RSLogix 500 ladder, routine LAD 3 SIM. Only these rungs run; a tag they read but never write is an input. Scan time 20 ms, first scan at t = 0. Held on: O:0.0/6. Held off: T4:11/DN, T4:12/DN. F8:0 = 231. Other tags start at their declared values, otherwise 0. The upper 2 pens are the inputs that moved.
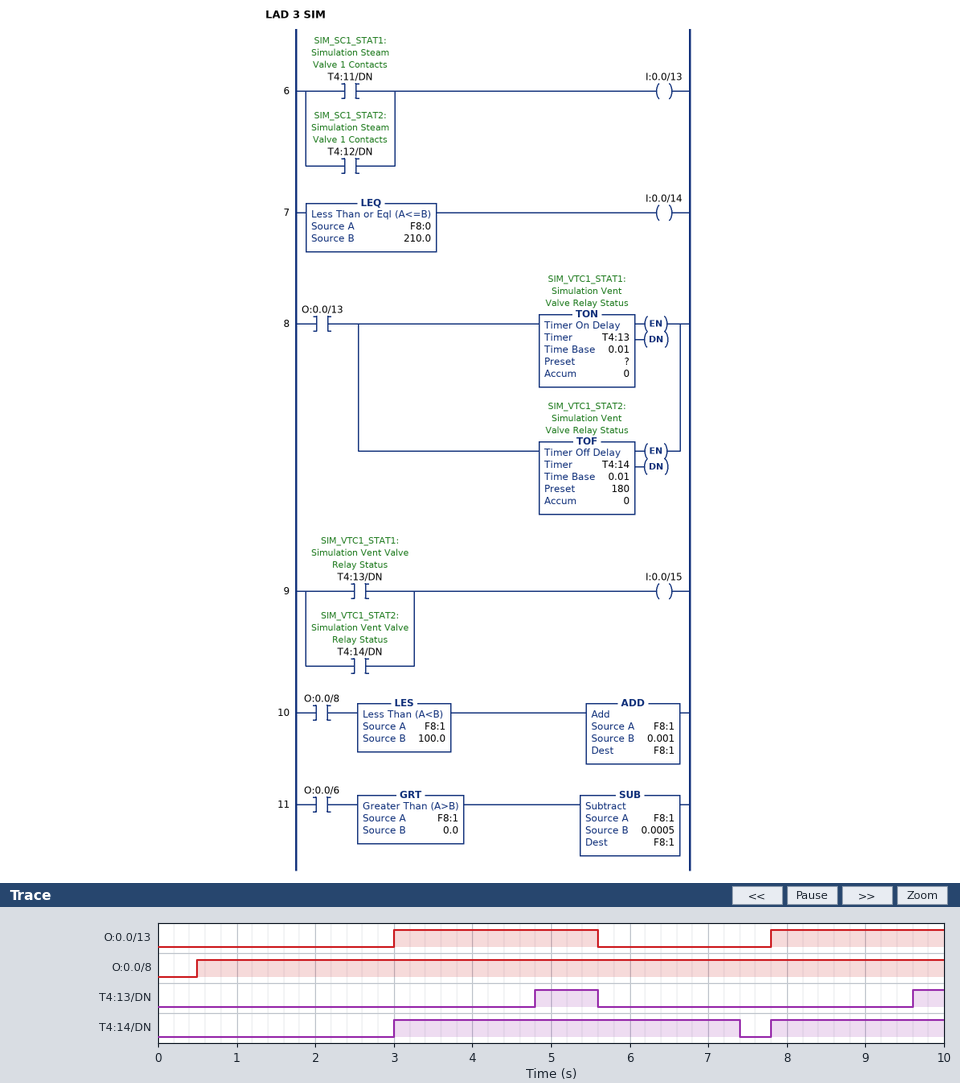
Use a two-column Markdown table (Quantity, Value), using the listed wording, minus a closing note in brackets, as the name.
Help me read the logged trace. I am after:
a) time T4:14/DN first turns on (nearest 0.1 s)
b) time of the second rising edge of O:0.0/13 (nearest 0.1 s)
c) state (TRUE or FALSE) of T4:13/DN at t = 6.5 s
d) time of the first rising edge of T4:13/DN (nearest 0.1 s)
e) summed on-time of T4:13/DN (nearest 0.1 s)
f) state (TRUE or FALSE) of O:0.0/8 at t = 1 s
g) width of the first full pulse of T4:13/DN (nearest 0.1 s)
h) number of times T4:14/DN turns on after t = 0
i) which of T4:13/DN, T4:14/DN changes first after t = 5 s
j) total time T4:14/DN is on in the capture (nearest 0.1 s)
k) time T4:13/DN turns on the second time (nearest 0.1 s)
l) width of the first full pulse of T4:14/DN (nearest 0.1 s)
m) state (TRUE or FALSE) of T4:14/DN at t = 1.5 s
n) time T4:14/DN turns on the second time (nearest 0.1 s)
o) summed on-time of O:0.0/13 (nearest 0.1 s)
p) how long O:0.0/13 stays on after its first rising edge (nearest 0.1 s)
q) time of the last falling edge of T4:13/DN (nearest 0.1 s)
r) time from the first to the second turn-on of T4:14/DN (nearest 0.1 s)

| Quantity | Value |
|---|---|
| time T4:14/DN first turns on | 3.0 s |
| time of the second rising edge of O:0.0/13 | 7.8 s |
| state (TRUE or FALSE) of T4:13/DN at t = 6.5 s | FALSE |
| time of the first rising edge of T4:13/DN | 4.8 s |
| summed on-time of T4:13/DN | 1.2 s |
| state (TRUE or FALSE) of O:0.0/8 at t = 1 s | TRUE |
| width of the first full pulse of T4:13/DN | 0.8 s |
| number of times T4:14/DN turns on after t = 0 | 2 |
| which of T4:13/DN, T4:14/DN changes first after t = 5 s | T4:13/DN |
| total time T4:14/DN is on in the capture | 6.6 s |
| time T4:13/DN turns on the second time | 9.6 s |
| width of the first full pulse of T4:14/DN | 4.4 s |
| state (TRUE or FALSE) of T4:14/DN at t = 1.5 s | FALSE |
| time T4:14/DN turns on the second time | 7.8 s |
| summed on-time of O:0.0/13 | 4.8 s |
| how long O:0.0/13 stays on after its first rising edge | 2.6 s |
| time of the last falling edge of T4:13/DN | 5.6 s |
| time from the first to the second turn-on of T4:14/DN | 4.8 s |
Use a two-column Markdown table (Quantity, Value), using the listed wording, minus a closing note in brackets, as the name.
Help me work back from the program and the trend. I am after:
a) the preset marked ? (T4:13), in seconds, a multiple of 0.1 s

| Quantity | Value |
|---|---|
| the preset marked ? (T4:13), in seconds, a multiple of 0.1 s | 1.8 s |
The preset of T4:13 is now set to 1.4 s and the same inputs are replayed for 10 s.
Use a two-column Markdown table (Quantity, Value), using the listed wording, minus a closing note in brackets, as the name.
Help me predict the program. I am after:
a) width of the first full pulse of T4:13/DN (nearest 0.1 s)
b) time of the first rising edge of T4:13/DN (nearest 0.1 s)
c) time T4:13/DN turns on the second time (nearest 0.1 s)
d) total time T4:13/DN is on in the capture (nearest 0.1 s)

| Quantity | Value |
|---|---|
| width of the first full pulse of T4:13/DN | 1.2 s |
| time of the first rising edge of T4:13/DN | 4.4 s |
| time T4:13/DN turns on the second time | 9.2 s |
| total time T4:13/DN is on in the capture | 2.0 s |
